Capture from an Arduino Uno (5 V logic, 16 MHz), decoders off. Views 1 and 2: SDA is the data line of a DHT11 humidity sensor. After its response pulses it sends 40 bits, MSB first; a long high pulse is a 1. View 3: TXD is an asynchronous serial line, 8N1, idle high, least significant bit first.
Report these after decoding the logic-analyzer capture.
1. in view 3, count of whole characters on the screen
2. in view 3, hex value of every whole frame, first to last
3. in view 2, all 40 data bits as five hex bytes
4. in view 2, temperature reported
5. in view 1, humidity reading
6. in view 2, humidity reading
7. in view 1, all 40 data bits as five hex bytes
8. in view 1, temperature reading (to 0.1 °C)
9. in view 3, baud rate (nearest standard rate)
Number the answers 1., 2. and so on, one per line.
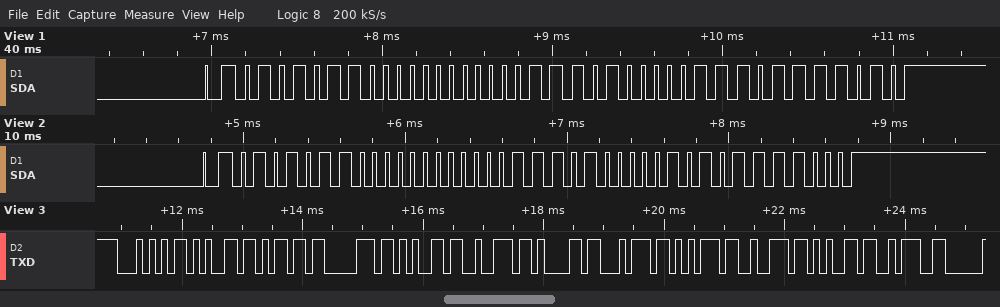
1. 12
2. 54 65 6D 70 65 72 61 74 75 72 65 3A
3. 56 00 1D 05 78
4. 29.5 °C
5. 86 %
6. 86 %
7. 56 00 1D 07 7A
8. 29.7 °C
9. 9600 baud
